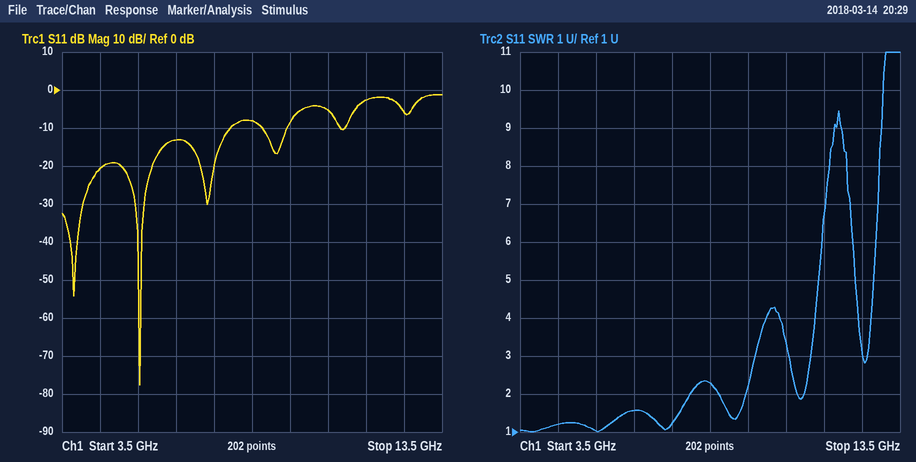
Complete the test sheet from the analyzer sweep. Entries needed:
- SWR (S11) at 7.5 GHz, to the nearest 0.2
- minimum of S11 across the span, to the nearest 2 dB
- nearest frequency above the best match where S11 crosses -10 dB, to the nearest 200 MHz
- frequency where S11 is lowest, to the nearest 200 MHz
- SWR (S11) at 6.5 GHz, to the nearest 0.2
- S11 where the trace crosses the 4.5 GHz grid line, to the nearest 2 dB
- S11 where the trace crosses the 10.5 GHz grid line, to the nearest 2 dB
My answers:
1.2
-78 dB
8.0 GHz
5.6 GHz
1.6
-20 dB
-6 dB
